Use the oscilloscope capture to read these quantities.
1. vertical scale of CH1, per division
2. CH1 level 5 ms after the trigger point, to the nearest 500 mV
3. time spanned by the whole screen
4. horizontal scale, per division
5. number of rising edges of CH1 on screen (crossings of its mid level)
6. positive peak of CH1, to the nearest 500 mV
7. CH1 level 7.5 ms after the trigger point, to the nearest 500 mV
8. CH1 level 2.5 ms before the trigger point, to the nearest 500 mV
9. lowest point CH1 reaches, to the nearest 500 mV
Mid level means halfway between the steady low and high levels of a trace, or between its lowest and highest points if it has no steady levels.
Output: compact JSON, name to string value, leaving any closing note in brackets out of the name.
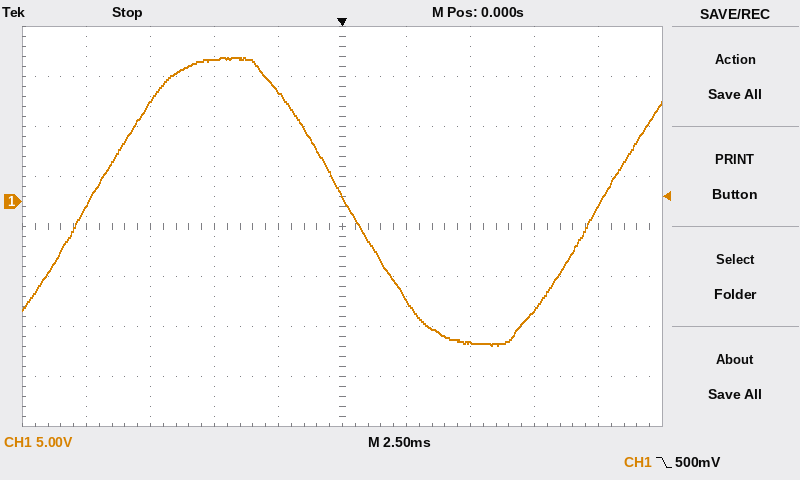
{"vertical scale of CH1, per division": "5 V", "CH1 level 5 ms after the trigger point, to the nearest 500 mV": "-14.0 V", "time spanned by the whole screen": "25 ms", "horizontal scale, per division": "2.5 ms", "number of rising edges of CH1 on screen": "2", "positive peak of CH1, to the nearest 500 mV": "14.5 V", "CH1 level 7.5 ms after the trigger point, to the nearest 500 mV": "-11.0 V", "CH1 level 2.5 ms before the trigger point, to the nearest 500 mV": "11.0 V", "lowest point CH1 reaches, to the nearest 500 mV": "-14.5 V"}
